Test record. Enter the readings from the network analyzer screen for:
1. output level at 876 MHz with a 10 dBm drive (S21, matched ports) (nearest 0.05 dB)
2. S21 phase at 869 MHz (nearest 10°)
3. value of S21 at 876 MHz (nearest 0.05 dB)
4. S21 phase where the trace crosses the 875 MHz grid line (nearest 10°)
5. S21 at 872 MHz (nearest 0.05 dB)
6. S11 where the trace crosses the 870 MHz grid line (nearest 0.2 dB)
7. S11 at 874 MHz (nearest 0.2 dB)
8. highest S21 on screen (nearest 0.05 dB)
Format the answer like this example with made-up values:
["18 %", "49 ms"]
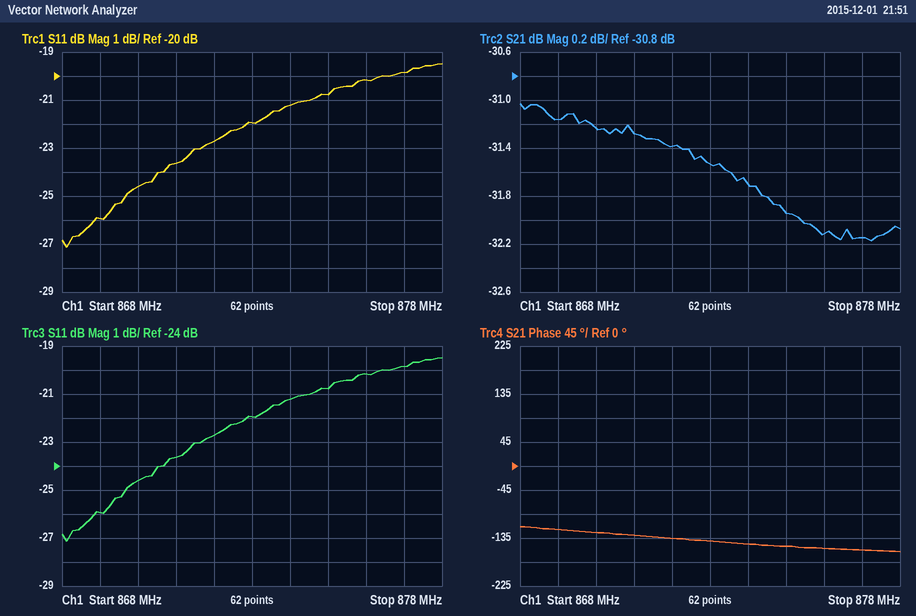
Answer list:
["-22.10 dBm", "-120°", "-32.10 dB", "-150°", "-31.40 dB", "-24.6 dB", "-21.2 dB", "-31.05 dB"]
